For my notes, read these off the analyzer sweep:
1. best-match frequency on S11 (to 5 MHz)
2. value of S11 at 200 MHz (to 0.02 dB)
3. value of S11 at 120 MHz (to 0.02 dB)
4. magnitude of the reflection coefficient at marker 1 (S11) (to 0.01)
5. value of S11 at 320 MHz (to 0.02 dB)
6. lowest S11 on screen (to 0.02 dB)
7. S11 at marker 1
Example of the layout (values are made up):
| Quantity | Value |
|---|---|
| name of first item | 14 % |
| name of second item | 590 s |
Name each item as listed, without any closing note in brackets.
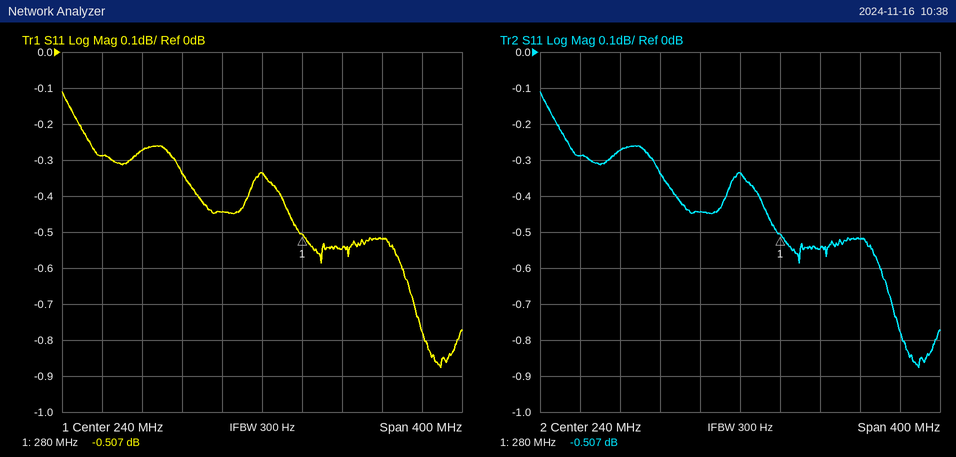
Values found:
| Quantity | Value |
|---|---|
| best-match frequency on S11 | 420 MHz |
| value of S11 at 200 MHz | -0.44 dB |
| value of S11 at 120 MHz | -0.28 dB |
| magnitude of the reflection coefficient at marker 1 (S11) | 0.94 |
| value of S11 at 320 MHz | -0.54 dB |
| lowest S11 on screen | -0.88 dB |
| S11 at marker 1 | -0.507 dB |
